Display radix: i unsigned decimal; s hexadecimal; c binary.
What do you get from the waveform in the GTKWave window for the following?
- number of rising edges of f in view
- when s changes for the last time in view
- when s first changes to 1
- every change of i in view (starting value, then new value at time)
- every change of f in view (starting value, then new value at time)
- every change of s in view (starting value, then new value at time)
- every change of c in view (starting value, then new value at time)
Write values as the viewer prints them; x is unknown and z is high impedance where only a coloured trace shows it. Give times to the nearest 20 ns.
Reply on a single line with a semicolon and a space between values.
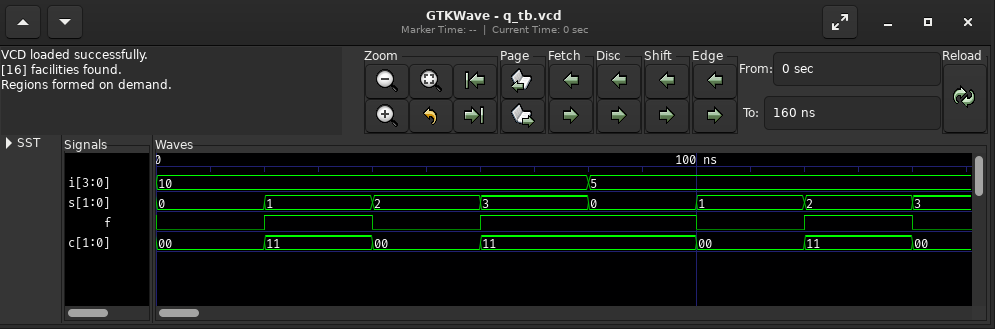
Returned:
3; 140 ns; 20 ns; 10, 5 at 80 ns; 0, 1 at 20 ns, 0 at 40 ns, 1 at 60 ns, 0 at 100 ns, 1 at 120 ns, 0 at 140 ns; 0, 1 at 20 ns, 2 at 40 ns, 3 at 60 ns, 0 at 80 ns, 1 at 100 ns, 2 at 120 ns, 3 at 140 ns; 00, 11 at 20 ns, 00 at 40 ns, 11 at 60 ns, 00 at 100 ns, 11 at 120 ns, 00 at 140 ns
